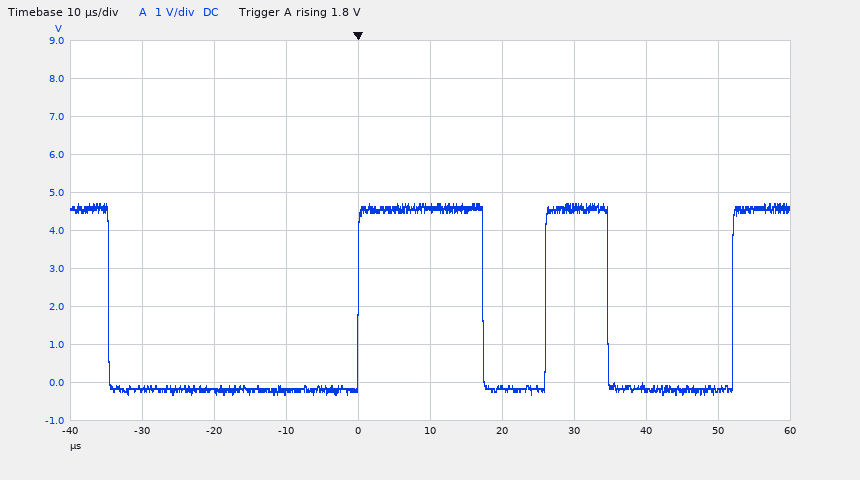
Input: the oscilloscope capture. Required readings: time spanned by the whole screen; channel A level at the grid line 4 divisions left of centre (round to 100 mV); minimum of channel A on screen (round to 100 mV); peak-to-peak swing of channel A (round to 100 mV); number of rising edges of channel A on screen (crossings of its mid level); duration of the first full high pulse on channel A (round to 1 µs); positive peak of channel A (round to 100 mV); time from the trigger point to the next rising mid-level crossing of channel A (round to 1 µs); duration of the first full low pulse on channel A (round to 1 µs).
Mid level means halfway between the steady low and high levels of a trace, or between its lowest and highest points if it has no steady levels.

100 µs
-200 mV
-300 mV
5.0 V
3
17 µs
4.7 V
26 µs
35 µs
